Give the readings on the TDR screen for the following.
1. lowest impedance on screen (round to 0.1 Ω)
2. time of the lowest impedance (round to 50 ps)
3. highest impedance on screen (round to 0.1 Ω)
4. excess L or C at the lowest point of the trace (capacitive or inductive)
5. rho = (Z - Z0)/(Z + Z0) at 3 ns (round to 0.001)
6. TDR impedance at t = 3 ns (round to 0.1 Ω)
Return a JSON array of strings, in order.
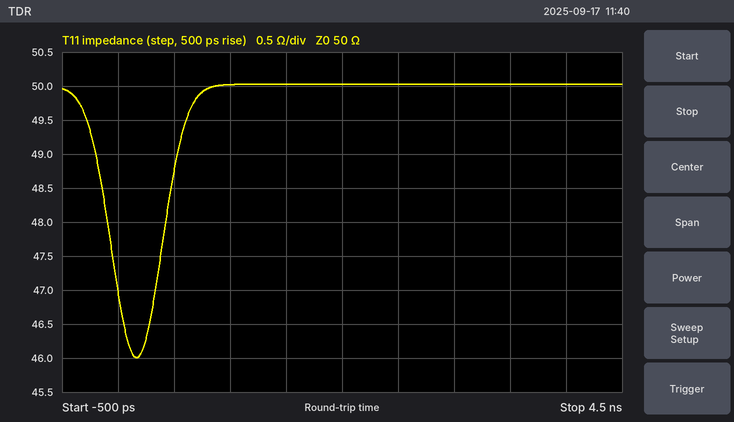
["46.0 Ω", "150 ps", "50.0 Ω", "capacitive", "0.000", "50.0 Ω"]
